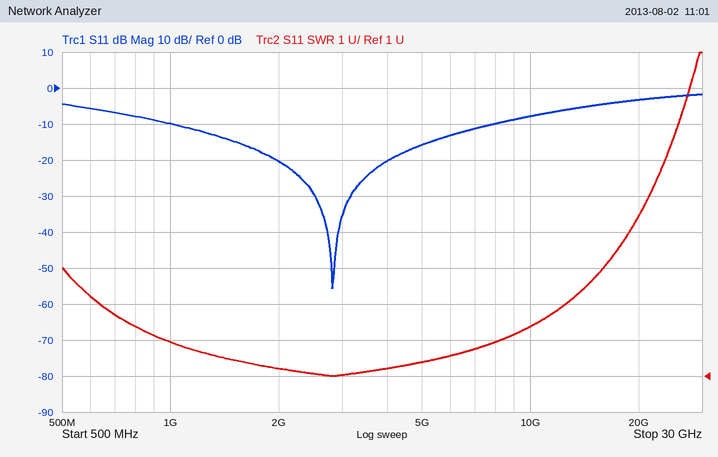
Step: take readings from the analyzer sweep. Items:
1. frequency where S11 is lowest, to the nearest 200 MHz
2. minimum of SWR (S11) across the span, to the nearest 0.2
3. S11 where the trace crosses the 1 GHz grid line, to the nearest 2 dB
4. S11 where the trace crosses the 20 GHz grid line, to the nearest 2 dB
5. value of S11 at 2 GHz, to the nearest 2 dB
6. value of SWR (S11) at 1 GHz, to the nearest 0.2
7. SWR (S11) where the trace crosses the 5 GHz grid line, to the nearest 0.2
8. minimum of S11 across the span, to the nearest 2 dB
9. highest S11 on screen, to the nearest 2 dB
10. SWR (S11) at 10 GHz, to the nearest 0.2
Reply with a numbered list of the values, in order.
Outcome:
1. 2.8 GHz
2. 1.0
3. -10 dB
4. -4 dB
5. -20 dB
6. 2.0
7. 1.4
8. -56 dB
9. -2 dB
10. 2.4
